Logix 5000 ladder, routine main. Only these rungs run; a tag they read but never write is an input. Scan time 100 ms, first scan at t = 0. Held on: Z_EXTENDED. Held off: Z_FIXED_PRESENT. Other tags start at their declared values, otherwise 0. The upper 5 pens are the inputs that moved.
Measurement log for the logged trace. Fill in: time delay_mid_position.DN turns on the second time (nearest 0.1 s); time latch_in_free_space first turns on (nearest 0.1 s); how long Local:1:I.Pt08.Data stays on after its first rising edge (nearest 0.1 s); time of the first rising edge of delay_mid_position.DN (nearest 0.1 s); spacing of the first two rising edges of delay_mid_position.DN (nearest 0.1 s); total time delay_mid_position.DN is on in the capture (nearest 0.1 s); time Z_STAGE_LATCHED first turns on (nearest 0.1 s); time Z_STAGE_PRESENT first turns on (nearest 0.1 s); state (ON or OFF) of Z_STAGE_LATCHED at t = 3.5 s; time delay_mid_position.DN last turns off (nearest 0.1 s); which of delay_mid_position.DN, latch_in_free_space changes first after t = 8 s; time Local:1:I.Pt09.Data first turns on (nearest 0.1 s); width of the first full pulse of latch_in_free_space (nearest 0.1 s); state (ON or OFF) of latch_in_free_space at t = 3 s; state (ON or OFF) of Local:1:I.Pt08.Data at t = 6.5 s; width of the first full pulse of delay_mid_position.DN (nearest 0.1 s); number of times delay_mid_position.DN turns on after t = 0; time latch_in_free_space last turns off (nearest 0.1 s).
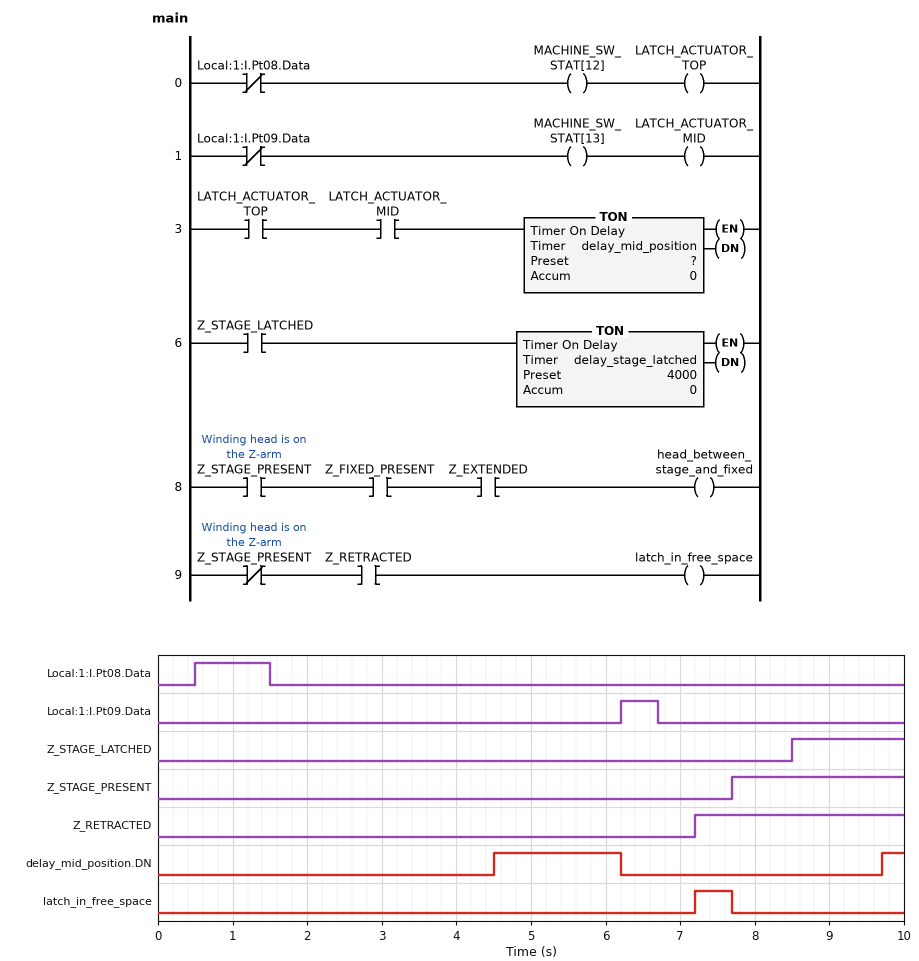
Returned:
9.7 s
7.2 s
1.0 s
4.5 s
5.2 s
2.0 s
8.5 s
7.7 s
OFF
6.2 s
delay_mid_position.DN
6.2 s
0.5 s
OFF
OFF
1.7 s
2
7.7 s
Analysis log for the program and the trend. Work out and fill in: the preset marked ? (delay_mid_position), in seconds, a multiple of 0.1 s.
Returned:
3.0 s
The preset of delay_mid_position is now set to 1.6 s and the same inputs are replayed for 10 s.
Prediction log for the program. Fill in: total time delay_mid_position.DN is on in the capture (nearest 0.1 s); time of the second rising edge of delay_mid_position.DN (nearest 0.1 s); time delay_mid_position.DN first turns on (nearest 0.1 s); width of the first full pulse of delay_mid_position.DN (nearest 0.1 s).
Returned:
4.8 s
8.3 s
3.1 s
3.1 s
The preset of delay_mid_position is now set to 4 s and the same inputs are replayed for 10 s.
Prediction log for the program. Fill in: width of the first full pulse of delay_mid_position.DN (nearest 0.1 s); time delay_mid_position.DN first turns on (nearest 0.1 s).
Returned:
0.7 s
5.5 s
